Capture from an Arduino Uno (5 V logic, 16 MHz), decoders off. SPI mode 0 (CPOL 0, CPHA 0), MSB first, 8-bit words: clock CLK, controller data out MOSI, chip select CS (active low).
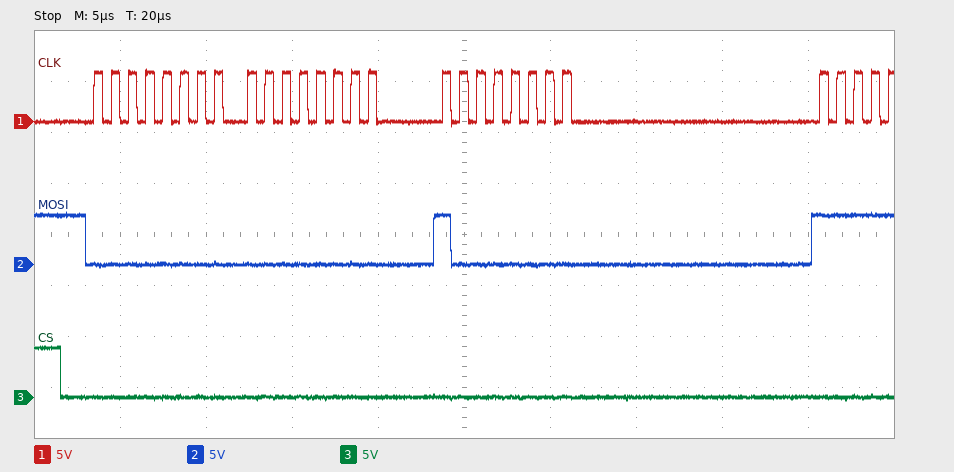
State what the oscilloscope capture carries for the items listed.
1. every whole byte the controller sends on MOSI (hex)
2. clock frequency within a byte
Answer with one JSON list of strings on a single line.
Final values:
["00 00 80", "1 MHz"]
